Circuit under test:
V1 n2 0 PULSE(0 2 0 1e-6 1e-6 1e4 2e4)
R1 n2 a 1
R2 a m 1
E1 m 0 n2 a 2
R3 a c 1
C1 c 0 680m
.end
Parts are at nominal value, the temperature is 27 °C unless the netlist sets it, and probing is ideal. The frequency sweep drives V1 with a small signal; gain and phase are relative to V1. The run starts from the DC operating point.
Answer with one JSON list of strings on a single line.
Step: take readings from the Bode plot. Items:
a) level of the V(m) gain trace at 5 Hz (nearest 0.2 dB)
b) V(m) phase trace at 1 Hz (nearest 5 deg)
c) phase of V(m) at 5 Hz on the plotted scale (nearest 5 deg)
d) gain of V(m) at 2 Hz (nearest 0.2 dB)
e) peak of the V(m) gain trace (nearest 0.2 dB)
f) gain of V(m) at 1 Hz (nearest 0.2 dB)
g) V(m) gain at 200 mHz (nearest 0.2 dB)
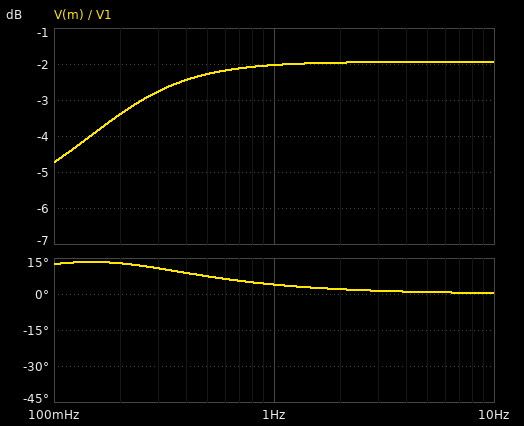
["-2.0 dB", "5 deg", "0 deg", "-2.0 dB", "-2.0 dB", "-2.0 dB", "-3.4 dB"]
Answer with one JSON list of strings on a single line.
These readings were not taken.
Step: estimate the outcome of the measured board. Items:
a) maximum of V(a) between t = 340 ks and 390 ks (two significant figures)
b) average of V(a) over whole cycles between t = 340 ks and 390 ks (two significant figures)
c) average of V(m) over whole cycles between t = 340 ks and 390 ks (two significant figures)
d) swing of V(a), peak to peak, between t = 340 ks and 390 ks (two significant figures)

["1.5 V", "750 mV", "500 mV", "1.5 V"]
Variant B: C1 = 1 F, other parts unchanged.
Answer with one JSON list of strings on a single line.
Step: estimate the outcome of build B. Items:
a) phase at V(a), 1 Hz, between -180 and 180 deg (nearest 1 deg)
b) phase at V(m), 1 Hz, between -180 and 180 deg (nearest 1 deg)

["-2 deg", "3 deg"]
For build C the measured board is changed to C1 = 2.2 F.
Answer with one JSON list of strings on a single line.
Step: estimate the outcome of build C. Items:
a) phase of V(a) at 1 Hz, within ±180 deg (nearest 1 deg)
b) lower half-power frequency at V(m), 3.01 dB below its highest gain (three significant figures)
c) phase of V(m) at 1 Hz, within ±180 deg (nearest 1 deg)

["-1 deg", "27.1 mHz", "1 deg"]
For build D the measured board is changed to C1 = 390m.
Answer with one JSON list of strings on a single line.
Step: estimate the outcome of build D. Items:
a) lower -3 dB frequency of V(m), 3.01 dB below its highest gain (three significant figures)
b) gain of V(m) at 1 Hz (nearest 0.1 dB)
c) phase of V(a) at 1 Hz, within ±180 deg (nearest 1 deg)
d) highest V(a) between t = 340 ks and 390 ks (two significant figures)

["153 mHz", "-2.2 dB", "-4 deg", "1.5 V"]
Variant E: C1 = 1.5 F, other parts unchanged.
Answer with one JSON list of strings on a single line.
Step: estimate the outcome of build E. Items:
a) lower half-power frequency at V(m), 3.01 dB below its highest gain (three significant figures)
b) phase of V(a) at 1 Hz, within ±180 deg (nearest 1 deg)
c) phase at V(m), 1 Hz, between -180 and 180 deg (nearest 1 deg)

["39.7 mHz", "-1 deg", "2 deg"]
